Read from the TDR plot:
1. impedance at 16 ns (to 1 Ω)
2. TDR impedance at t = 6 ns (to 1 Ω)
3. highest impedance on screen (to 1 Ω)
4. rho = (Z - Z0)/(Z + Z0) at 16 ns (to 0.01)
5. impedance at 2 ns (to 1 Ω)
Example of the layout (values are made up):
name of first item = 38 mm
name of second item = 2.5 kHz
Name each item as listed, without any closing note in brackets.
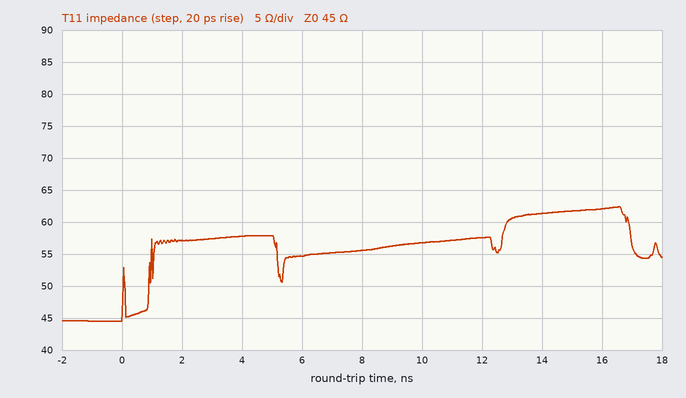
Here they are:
impedance at 16 ns = 62 Ω
TDR impedance at t = 6 ns = 55 Ω
highest impedance on screen = 62 Ω
rho = (Z - Z0)/(Z + Z0) at 16 ns = +0.16
impedance at 2 ns = 57 Ω
